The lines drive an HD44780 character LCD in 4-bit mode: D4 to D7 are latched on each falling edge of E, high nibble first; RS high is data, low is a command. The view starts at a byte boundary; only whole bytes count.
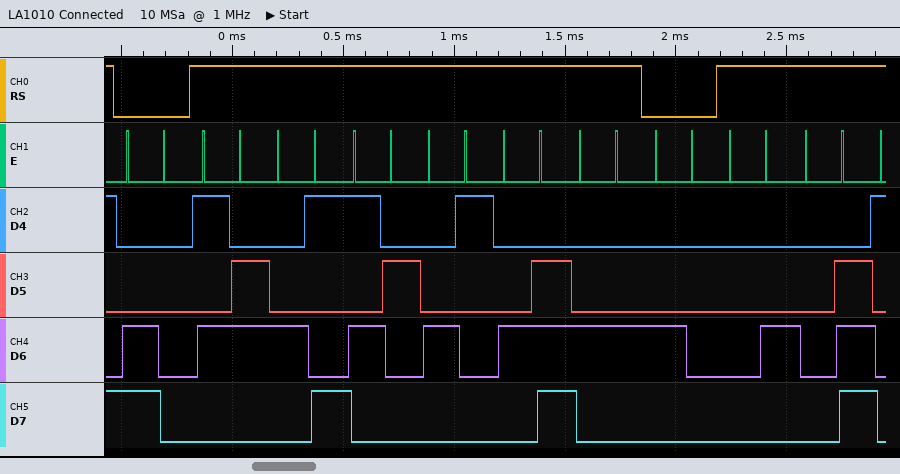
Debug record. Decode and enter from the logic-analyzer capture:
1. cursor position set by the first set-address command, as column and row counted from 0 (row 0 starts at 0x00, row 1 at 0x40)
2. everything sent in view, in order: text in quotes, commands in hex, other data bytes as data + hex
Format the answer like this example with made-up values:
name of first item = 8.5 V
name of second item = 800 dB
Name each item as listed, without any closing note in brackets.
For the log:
cursor position set by the first set-address command, as column and row counted from 0 = column 0, row 1
everything sent in view, in order: text in quotes, commands in hex, other data bytes as data + hex = 0xC0 "VIRAND" 0x40 data 04 0E
